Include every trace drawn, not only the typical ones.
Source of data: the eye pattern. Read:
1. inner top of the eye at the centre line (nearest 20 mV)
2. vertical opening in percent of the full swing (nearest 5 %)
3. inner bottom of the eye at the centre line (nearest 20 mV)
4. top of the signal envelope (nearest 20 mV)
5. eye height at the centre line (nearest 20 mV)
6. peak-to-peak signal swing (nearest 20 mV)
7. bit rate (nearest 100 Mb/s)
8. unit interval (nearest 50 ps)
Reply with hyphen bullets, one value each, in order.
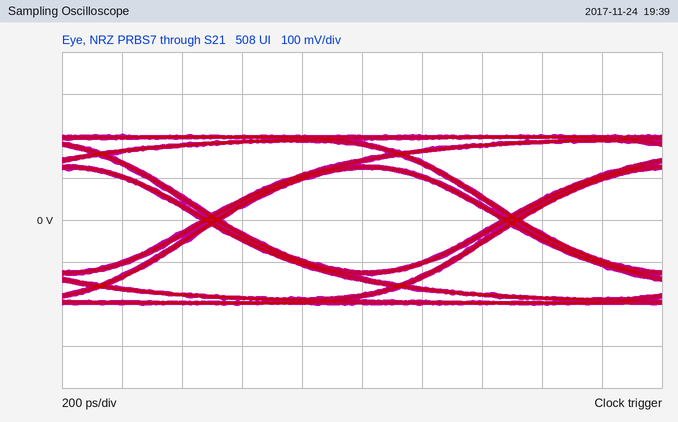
- 120 mV
- 60 %
- -120 mV
- 200 mV
- 240 mV
- 400 mV
- 1.0 Gb/s
- 1.00 ns
